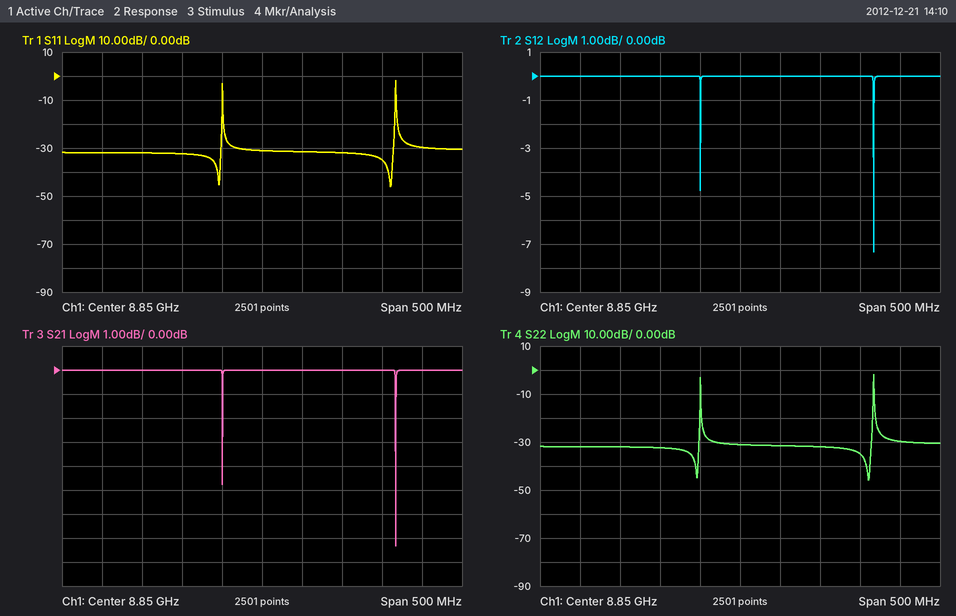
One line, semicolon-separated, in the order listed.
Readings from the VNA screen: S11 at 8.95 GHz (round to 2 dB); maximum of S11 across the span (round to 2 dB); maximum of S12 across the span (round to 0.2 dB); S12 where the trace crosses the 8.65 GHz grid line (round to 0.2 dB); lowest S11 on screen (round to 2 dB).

-32 dB; -2 dB; 0.0 dB; 0.0 dB; -46 dB
